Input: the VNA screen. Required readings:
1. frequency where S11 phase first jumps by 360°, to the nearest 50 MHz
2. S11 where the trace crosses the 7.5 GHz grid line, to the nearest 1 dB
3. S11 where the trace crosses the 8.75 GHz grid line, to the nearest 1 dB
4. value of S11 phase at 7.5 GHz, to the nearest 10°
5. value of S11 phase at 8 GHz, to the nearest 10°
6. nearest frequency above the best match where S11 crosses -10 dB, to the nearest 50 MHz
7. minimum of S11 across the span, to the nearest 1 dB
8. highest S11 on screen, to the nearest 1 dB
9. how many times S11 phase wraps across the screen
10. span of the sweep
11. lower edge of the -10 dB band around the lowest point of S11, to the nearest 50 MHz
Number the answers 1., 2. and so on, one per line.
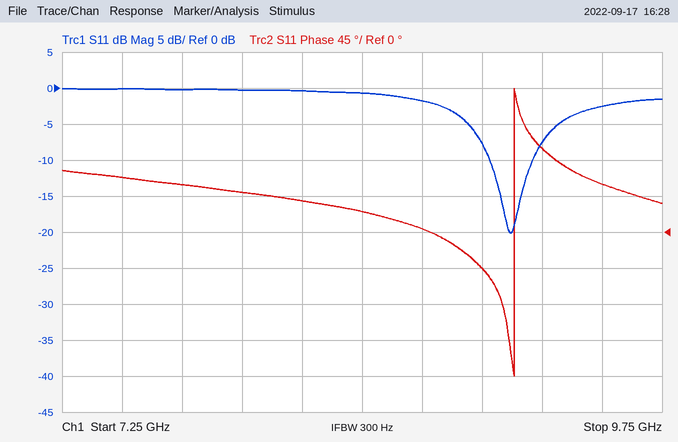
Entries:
1. 9.15 GHz
2. 0 dB
3. -2 dB
4. 70°
5. 50°
6. 9.20 GHz
7. -20 dB
8. 0 dB
9. 1
10. 2.5 GHz
11. 9.05 GHz
